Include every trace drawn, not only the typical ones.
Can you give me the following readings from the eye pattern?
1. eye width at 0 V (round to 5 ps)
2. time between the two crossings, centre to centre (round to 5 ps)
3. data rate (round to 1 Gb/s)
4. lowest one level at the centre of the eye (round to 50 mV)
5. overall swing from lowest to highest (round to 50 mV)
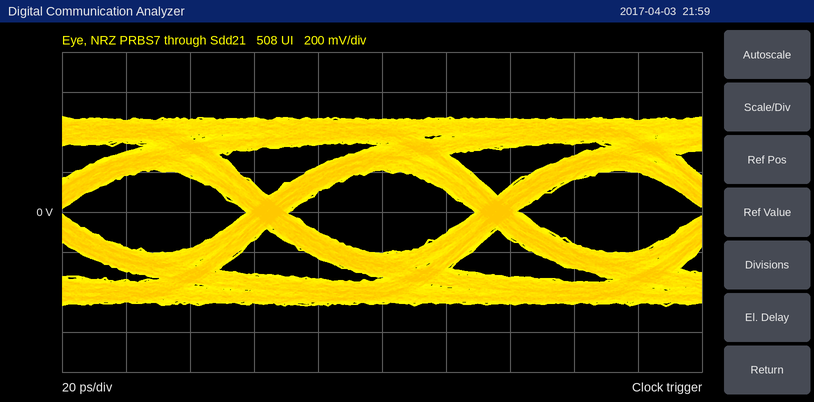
60 ps
70 ps
14 Gb/s
200 mV
950 mV
